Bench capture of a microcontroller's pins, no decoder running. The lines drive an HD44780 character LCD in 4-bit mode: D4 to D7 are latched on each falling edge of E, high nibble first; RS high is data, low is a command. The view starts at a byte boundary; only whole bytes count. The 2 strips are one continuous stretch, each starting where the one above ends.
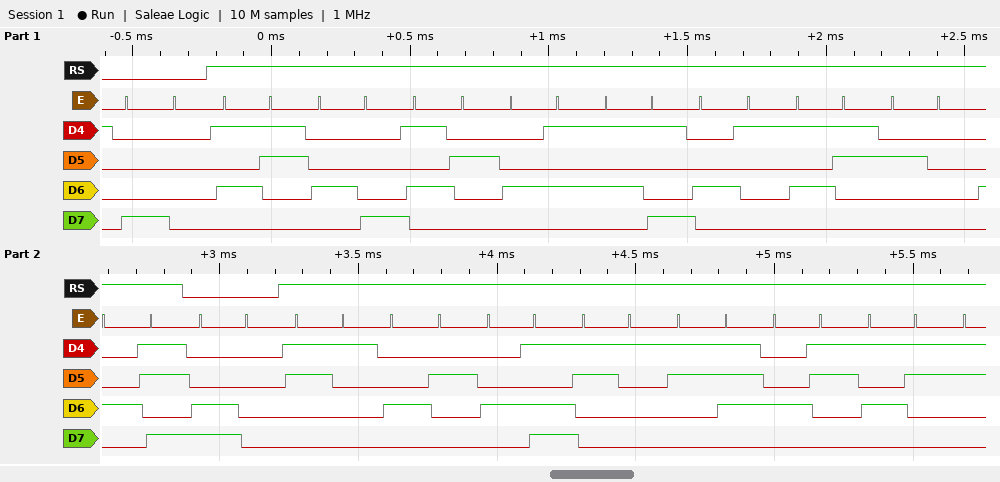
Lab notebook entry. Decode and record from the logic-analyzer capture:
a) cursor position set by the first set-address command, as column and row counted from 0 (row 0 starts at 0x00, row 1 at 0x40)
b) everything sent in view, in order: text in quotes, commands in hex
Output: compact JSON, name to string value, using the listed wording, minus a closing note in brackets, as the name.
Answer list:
{"cursor position set by the first set-address command, as column and row counted from 0": "column 0, row 0", "everything sent in view, in order: text in quotes, commands in hex": "0x80 \"SHREYAS K\" 0xC0 \"1BM17CS\""}
